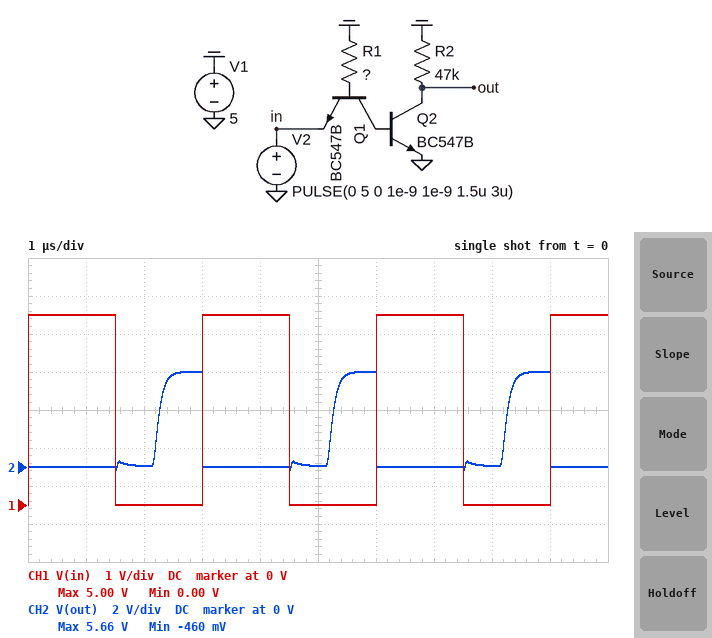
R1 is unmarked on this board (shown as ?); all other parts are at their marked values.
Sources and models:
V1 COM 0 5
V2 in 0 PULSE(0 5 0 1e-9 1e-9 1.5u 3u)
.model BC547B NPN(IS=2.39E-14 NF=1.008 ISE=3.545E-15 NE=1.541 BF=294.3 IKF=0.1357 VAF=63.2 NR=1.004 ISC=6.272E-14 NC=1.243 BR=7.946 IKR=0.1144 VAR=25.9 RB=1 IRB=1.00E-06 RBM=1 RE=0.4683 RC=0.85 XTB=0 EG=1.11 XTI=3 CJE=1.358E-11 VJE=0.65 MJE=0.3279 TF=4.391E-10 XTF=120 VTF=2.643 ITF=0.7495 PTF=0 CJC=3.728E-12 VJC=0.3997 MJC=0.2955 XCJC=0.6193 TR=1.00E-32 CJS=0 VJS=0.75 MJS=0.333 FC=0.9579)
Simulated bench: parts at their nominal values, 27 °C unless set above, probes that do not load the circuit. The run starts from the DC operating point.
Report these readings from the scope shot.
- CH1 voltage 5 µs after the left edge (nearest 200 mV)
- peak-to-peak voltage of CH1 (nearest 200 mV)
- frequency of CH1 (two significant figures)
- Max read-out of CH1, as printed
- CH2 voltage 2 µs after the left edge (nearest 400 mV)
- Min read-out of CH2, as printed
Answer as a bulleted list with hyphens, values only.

- 0 V
- 5.0 V
- 330 kHz
- 5.00 V
- 0 V
- -460 mV
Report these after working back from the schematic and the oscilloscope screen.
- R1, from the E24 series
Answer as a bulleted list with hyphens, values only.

- 91 kΩ
